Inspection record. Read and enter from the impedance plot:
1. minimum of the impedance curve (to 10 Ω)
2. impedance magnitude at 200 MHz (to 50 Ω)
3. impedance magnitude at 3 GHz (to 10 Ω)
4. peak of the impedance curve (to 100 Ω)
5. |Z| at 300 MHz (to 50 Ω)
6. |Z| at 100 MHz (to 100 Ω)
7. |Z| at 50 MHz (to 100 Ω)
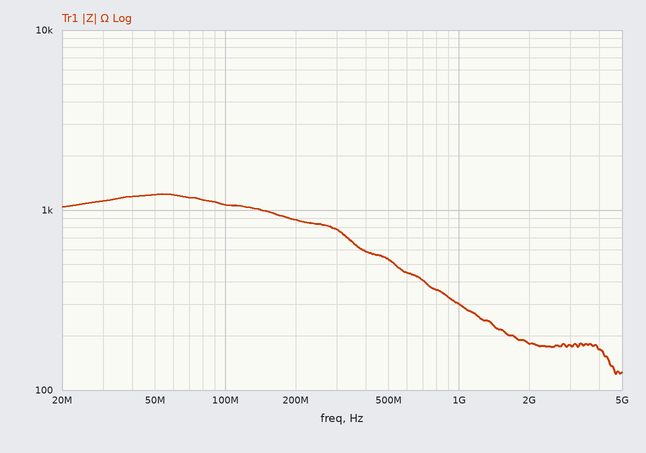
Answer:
120 Ω
900 Ω
180 Ω
1.2 kΩ
800 Ω
1.1 kΩ
1.2 kΩ
